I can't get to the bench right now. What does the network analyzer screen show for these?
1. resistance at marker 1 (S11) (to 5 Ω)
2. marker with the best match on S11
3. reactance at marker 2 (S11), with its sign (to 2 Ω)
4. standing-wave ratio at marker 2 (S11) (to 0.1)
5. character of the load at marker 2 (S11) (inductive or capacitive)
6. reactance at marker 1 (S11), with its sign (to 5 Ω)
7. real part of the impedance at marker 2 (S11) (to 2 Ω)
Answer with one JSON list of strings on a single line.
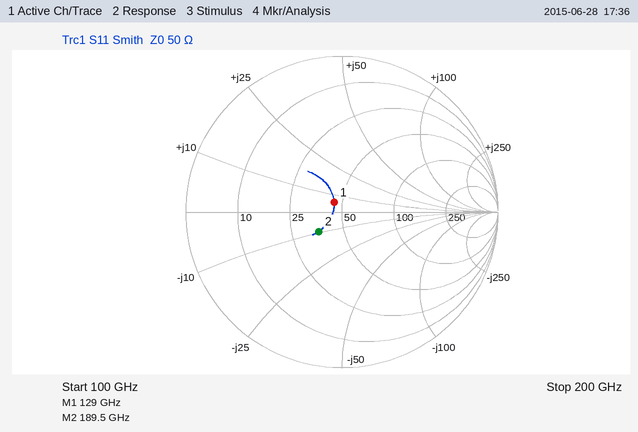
["45 Ω", "marker 1", "-10 Ω", "1.5", "capacitive", "+5 Ω", "36 Ω"]
